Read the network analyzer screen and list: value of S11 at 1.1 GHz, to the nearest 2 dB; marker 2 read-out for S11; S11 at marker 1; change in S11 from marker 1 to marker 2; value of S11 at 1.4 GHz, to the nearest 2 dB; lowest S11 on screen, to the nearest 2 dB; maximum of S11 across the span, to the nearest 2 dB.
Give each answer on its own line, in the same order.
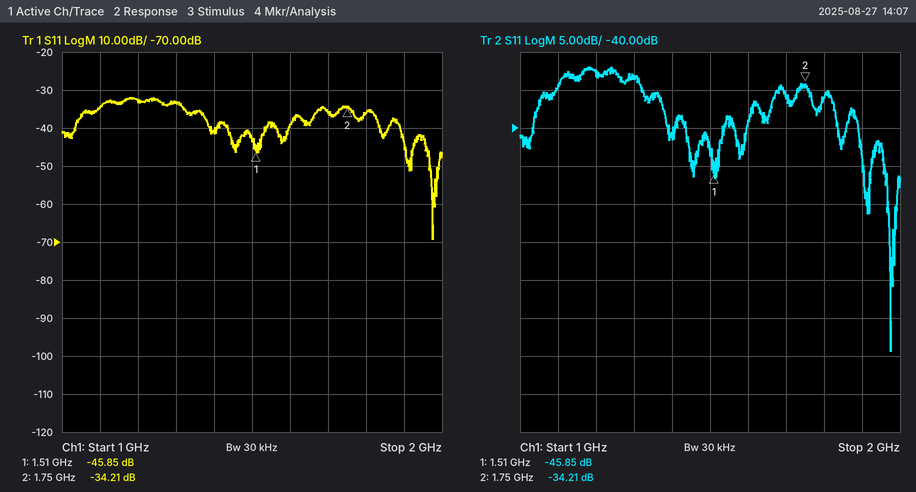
-34 dB
-34.21 dB
-45.85 dB
11.64 dB
-40 dB
-70 dB
-32 dB
